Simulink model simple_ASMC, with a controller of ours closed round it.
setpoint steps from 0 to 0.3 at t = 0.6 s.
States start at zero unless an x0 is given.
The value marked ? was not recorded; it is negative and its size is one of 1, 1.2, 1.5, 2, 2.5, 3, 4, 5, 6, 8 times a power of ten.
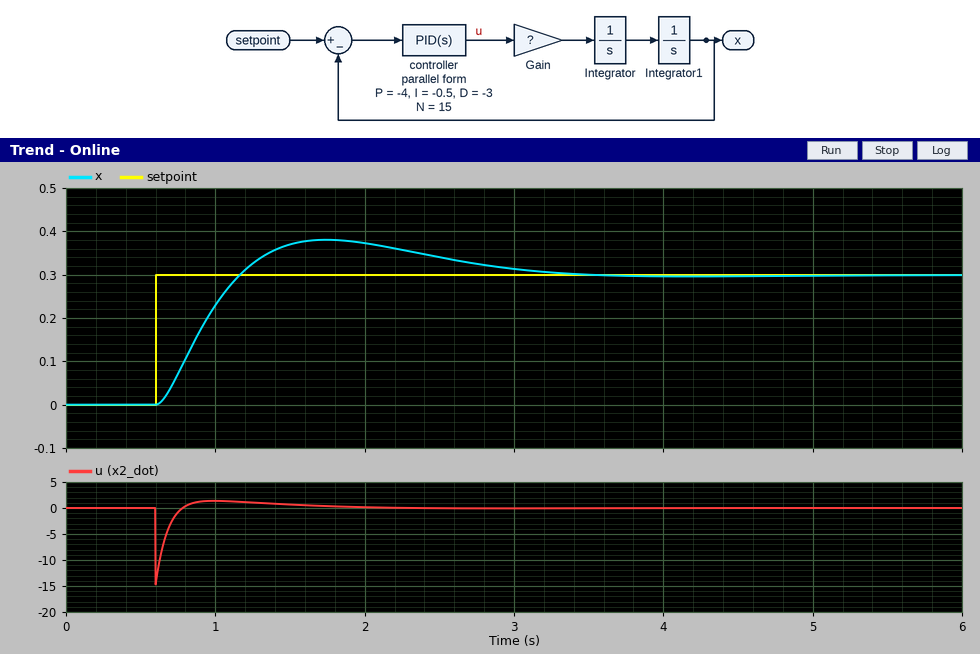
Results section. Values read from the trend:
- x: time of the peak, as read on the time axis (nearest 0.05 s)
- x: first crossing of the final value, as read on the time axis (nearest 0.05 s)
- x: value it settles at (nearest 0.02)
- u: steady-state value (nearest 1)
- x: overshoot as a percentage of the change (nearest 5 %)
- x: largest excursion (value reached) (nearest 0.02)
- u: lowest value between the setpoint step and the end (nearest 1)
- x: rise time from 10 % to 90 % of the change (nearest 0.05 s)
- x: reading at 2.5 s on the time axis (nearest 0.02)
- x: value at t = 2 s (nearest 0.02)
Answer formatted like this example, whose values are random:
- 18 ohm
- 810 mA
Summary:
- 1.75 s
- 1.15 s
- 0.30
- 0
- 25 %
- 0.38
- -15
- 0.40 s
- 0.34
- 0.38
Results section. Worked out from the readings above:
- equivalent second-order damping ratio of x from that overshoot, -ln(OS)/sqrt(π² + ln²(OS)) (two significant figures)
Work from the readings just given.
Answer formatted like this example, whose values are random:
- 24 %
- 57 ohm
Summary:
- 0.40
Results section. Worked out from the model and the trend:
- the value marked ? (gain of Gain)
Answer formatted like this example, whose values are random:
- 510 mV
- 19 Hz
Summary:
- -0.8
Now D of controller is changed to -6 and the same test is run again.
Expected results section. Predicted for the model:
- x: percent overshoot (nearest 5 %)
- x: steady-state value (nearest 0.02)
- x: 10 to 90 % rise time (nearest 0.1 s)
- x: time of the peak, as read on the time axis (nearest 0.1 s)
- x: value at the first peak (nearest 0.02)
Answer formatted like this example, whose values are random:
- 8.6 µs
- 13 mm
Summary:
- 10 %
- 0.30
- 0.3 s
- 1.3 s
- 0.34
